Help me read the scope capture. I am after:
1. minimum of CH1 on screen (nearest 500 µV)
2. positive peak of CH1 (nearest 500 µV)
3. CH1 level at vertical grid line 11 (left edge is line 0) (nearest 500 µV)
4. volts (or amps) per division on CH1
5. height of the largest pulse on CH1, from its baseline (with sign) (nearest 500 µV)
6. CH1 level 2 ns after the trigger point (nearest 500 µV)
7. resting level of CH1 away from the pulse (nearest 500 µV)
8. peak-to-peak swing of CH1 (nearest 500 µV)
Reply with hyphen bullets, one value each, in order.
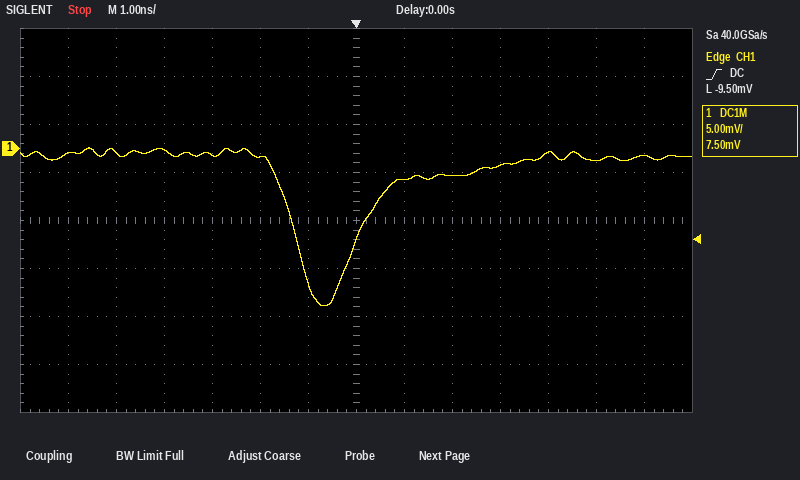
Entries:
- -16.5 mV
- 0.0 mV
- -500 µV
- 5 mV
- -15.5 mV
- -3.0 mV
- -1.0 mV
- 16.5 mV
